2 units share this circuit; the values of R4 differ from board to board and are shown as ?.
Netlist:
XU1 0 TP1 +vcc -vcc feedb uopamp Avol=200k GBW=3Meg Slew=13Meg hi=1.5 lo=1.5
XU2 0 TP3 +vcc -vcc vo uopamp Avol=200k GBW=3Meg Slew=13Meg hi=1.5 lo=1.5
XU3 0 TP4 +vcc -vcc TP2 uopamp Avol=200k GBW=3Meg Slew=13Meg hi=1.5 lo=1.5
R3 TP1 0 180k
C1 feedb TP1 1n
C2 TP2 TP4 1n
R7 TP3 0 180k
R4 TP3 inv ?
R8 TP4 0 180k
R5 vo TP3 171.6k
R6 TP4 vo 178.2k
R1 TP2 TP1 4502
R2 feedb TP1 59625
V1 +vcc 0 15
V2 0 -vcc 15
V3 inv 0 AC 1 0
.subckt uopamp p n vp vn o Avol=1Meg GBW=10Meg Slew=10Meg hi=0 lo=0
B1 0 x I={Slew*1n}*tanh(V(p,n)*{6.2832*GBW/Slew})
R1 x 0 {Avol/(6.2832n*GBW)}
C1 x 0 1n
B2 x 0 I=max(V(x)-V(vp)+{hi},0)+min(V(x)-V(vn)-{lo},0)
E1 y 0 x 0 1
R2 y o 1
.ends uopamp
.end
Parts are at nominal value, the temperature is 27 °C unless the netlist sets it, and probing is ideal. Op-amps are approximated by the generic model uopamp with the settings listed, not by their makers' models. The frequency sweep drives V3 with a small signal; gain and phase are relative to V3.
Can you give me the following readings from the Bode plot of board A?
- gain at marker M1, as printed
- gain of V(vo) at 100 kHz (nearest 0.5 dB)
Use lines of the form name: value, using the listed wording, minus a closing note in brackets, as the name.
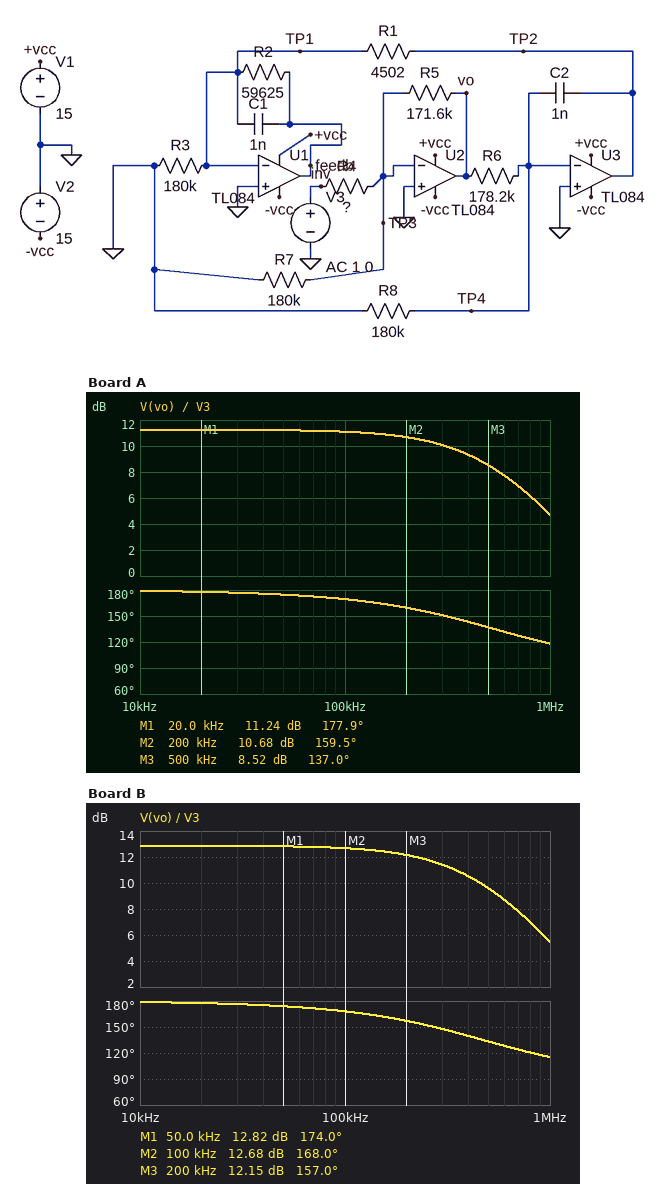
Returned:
gain at marker M1, as printed: 11.24 dB
gain of V(vo) at 100 kHz: 11.0 dB
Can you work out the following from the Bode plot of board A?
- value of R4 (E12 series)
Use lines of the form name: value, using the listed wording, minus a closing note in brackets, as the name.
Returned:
value of R4: 47 kΩ
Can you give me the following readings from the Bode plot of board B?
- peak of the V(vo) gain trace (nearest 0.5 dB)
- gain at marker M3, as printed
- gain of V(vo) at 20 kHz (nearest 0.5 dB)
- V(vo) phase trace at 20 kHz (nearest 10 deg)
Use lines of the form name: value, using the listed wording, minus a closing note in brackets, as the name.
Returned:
peak of the V(vo) gain trace: 13.0 dB
gain at marker M3, as printed: 12.15 dB
gain of V(vo) at 20 kHz: 13.0 dB
V(vo) phase trace at 20 kHz: 180 deg
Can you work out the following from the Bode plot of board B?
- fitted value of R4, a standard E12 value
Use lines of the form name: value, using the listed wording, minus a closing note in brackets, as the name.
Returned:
fitted value of R4, a standard E12 value: 39 kΩ
